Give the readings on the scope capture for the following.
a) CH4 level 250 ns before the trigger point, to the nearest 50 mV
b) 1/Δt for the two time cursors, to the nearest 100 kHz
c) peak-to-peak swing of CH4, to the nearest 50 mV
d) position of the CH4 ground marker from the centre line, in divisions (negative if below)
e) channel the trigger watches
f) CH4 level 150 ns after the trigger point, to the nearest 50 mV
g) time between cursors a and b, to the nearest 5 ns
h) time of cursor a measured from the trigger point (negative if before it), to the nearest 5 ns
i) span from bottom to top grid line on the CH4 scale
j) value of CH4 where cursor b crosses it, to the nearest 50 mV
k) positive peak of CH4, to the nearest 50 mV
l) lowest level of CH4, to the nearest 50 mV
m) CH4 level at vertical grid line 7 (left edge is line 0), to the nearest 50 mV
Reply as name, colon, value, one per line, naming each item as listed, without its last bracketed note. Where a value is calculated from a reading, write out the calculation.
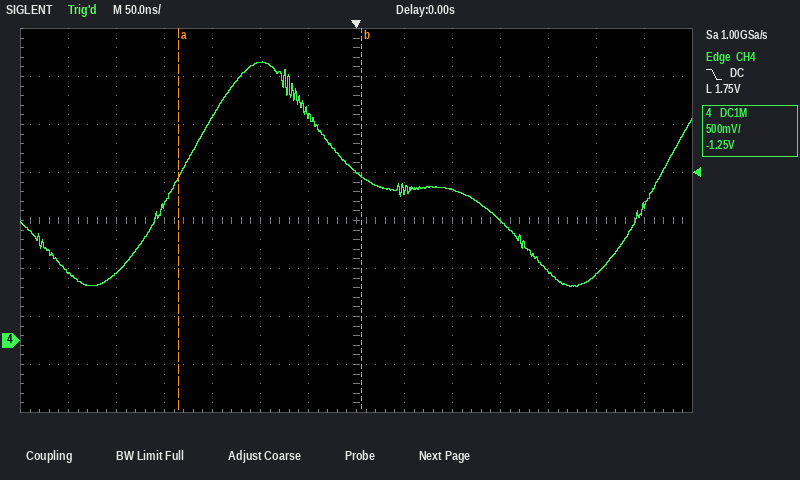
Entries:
CH4 level 250 ns before the trigger point, to the nearest 50 mV: 700 mV
1/Δt for the two time cursors, to the nearest 100 kHz: 1 / 190 ns ≈ 5.3 MHz
peak-to-peak swing of CH4, to the nearest 50 mV: 2.90 V − (550 mV) = 2.35 V
position of the CH4 ground marker from the centre line, in divisions: -2.5 div
channel the trigger watches: CH4
CH4 level 150 ns after the trigger point, to the nearest 50 mV: 1.25 V
time between cursors a and b, to the nearest 5 ns: 190 ns
time of cursor a measured from the trigger point (negative if before it), to the nearest 5 ns: -185 ns
span from bottom to top grid line on the CH4 scale: 4 V
value of CH4 where cursor b crosses it, to the nearest 50 mV: 1.70 V
positive peak of CH4, to the nearest 50 mV: 2.90 V
lowest level of CH4, to the nearest 50 mV: 550 mV
CH4 level at vertical grid line 7 (left edge is line 0), to the nearest 50 mV: 1.75 V
